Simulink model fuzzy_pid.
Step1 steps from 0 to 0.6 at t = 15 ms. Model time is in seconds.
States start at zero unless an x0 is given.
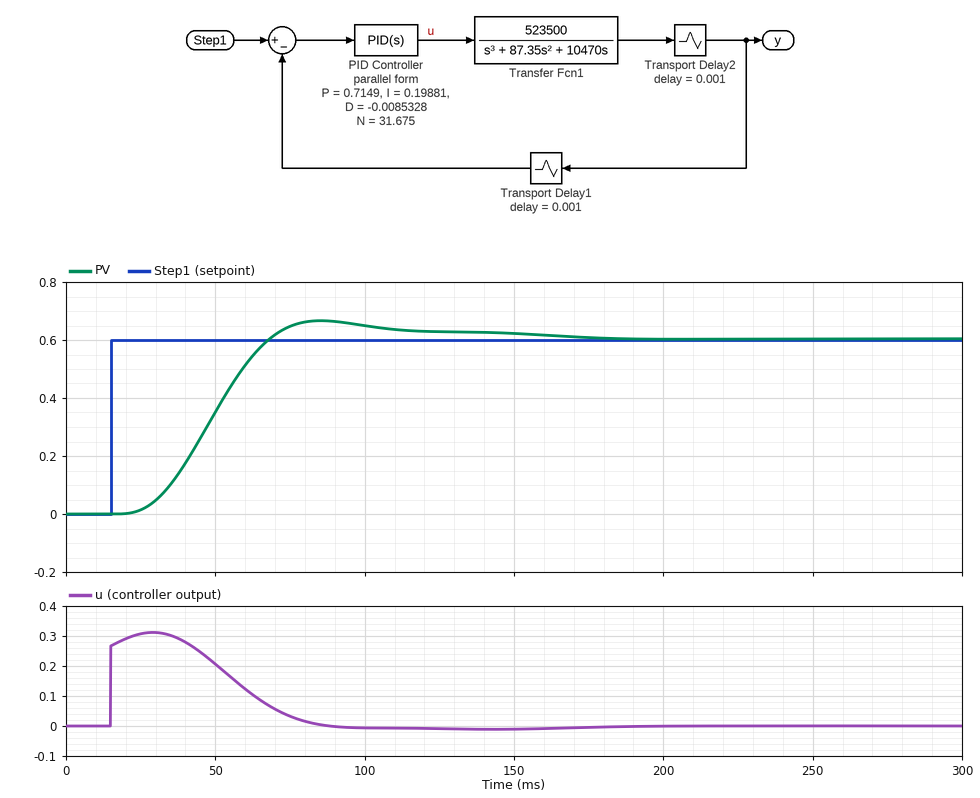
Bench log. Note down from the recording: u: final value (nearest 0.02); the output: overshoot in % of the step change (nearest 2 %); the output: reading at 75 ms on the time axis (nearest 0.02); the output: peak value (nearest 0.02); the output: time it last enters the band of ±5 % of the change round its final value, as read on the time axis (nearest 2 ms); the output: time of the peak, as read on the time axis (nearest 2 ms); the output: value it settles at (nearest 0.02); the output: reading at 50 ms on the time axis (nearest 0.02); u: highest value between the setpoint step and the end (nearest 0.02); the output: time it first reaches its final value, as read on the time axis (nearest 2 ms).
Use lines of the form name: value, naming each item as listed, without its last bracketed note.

u: final value: 0.00
the output: overshoot in % of the step change: 10 %
the output: reading at 75 ms on the time axis: 0.64
the output: peak value: 0.66
the output: time it last enters the band of ±5 % of the change round its final value, as read on the time axis: 114 ms
the output: time of the peak, as read on the time axis: 86 ms
the output: value it settles at: 0.60
the output: reading at 50 ms on the time axis: 0.36
u: highest value between the setpoint step and the end: 0.32
the output: time it first reaches its final value, as read on the time axis: 68 ms
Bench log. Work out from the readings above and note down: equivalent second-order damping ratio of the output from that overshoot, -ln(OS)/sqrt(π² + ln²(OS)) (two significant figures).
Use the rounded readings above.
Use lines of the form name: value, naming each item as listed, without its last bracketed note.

equivalent second-order damping ratio of the output from that overshoot, -ln(OS)/sqrt(π² + ln²(OS)): 0.59
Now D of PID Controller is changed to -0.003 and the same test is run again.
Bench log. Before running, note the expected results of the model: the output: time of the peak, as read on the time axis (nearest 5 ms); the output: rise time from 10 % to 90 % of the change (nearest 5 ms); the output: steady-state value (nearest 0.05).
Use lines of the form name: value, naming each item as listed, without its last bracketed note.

the output: time of the peak, as read on the time axis: 75 ms
the output: rise time from 10 % to 90 % of the change: 25 ms
the output: steady-state value: 0.60
